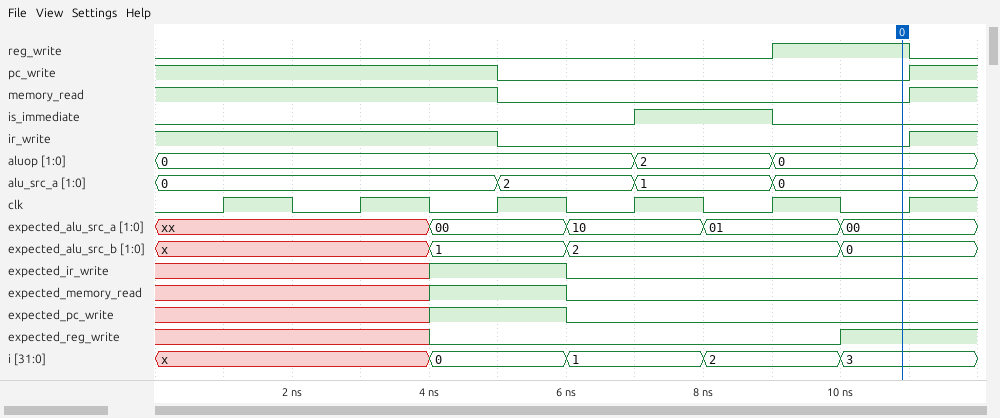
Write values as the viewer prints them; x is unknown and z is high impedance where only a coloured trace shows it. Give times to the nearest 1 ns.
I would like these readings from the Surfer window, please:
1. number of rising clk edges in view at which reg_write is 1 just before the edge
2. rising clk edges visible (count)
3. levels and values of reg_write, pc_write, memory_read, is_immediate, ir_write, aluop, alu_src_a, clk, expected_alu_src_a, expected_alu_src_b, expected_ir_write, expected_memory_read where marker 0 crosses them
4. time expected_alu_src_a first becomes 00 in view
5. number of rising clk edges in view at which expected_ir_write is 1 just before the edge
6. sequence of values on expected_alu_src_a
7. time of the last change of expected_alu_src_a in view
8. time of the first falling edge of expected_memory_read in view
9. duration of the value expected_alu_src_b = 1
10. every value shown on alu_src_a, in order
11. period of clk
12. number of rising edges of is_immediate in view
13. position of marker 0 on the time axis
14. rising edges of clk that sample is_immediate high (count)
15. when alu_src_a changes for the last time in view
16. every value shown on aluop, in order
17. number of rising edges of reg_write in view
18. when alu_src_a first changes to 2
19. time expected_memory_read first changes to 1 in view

1
6
reg_write=1, pc_write=0, memory_read=0, is_immediate=0, ir_write=0, aluop=0, alu_src_a=0, clk=0, expected_alu_src_a=00, expected_alu_src_b=0, expected_ir_write=0, expected_memory_read=0
4 ns
1
xx, 00, 10, 01, 00
10 ns
6 ns
2 ns
0, 2, 1, 0
2 ns
1
11 ns
1
9 ns
0, 2, 0
1
5 ns
4 ns
